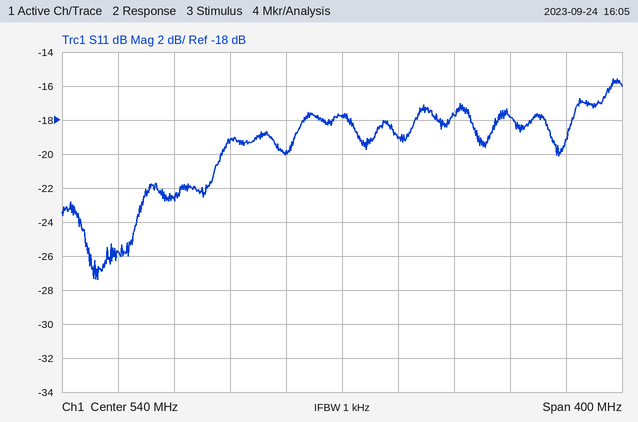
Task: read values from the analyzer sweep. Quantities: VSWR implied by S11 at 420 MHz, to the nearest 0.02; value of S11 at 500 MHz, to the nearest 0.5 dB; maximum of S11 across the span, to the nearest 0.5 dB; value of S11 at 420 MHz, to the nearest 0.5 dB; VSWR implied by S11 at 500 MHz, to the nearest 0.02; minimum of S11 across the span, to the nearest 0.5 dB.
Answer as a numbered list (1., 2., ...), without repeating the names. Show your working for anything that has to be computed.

1. |Γ| = 10^(-22.5/20) = 0.0750; VSWR = (1 + 0.0750)/(1 − 0.0750) ≈ 1.16
2. -20.0 dB
3. -15.5 dB
4. -22.5 dB
5. |Γ| = 10^(-20/20) = 0.1000; VSWR = (1 + 0.1000)/(1 − 0.1000) ≈ 1.22
6. -27.5 dB
